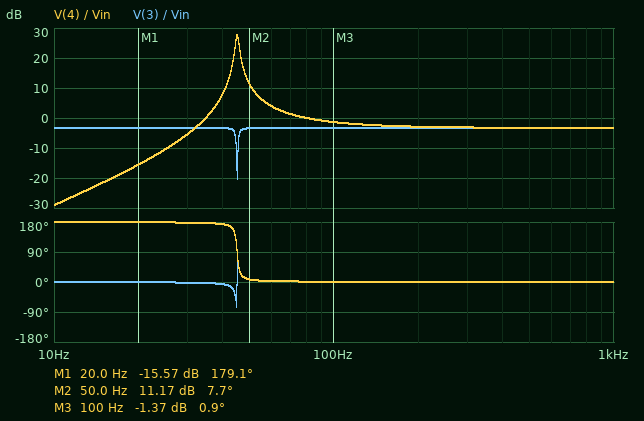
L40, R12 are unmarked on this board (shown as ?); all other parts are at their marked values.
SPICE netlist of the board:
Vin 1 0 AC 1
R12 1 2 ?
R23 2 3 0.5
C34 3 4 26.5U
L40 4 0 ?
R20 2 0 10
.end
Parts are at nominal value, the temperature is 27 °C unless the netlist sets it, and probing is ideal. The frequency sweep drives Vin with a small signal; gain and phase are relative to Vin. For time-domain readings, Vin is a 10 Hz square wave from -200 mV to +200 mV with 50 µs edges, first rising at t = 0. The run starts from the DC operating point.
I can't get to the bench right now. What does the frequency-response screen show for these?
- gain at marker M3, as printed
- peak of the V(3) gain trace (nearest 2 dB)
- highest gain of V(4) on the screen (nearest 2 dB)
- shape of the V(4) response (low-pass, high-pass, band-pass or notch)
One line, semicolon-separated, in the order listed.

-1.37 dB; -4 dB; 28 dB; high-pass
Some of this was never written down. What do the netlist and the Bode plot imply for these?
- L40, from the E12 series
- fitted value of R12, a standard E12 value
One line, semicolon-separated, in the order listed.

470 mH; 4.7 Ω
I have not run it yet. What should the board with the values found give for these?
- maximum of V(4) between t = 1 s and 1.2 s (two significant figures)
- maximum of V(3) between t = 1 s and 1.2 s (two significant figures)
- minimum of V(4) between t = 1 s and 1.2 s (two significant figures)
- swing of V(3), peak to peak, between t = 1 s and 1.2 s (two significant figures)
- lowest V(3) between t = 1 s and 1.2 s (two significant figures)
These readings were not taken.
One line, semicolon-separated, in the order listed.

210 mV; 140 mV; -210 mV; 280 mV; -140 mV
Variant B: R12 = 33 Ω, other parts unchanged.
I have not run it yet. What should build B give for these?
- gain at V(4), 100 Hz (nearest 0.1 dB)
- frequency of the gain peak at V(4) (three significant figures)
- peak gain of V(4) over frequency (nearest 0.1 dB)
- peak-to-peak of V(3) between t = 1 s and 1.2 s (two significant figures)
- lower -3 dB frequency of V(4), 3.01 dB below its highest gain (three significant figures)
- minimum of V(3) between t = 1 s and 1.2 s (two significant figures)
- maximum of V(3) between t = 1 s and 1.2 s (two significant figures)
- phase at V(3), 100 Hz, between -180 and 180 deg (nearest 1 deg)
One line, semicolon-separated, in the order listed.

-10.7 dB; 45.1 Hz; 11.6 dB; 100 mV; 43.8 Hz; -51 mV; 51 mV; 2 deg
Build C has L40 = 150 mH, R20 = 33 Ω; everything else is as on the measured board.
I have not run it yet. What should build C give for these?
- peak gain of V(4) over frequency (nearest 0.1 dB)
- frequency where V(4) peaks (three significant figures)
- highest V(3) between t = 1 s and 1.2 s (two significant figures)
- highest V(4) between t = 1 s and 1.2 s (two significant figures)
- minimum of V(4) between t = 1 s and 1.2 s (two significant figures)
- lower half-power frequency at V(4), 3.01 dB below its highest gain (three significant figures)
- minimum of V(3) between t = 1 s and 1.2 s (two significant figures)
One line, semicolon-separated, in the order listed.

23.1 dB; 79.9 Hz; 190 mV; 240 mV; -240 mV; 77.6 Hz; -190 mV
